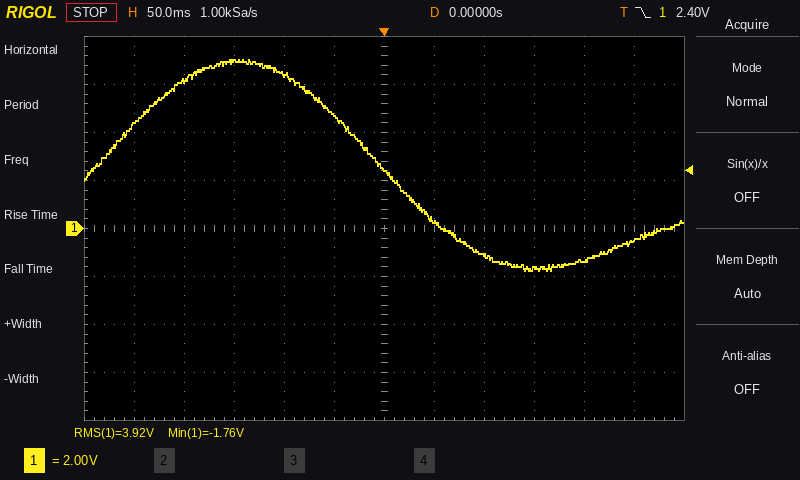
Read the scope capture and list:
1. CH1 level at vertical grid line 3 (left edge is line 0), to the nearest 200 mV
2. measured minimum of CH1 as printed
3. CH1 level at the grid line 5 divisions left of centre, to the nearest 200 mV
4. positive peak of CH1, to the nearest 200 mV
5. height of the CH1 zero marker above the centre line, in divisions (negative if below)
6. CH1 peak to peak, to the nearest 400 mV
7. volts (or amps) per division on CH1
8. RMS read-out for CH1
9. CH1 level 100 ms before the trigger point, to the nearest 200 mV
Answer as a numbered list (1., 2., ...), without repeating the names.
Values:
1. 7.0 V
2. -1.76 V
3. 4.4 V
4. 7.0 V
5. 0.0 div
6. 8.8 V
7. 2 V
8. 3.92 V
9. 6.4 V
